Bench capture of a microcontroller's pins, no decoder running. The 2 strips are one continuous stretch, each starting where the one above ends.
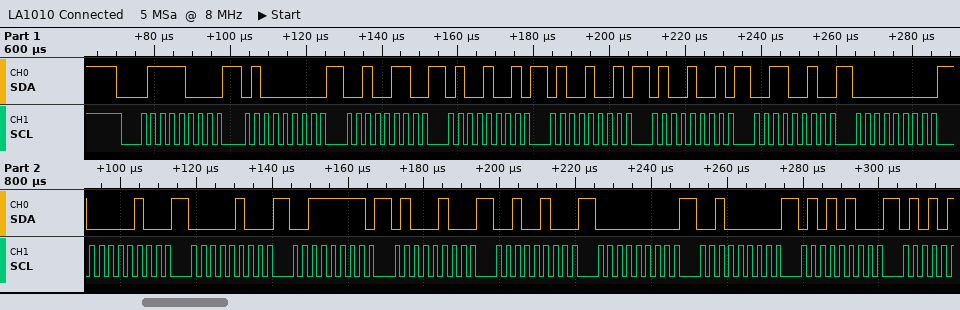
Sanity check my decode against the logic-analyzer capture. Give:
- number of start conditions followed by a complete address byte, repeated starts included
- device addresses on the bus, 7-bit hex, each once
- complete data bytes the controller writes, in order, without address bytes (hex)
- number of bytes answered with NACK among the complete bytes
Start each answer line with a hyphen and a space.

- 1
- 0x3C
- 40 26 49 49 49 32 00 04 04 3F 44 24 00 20 54
- 0
